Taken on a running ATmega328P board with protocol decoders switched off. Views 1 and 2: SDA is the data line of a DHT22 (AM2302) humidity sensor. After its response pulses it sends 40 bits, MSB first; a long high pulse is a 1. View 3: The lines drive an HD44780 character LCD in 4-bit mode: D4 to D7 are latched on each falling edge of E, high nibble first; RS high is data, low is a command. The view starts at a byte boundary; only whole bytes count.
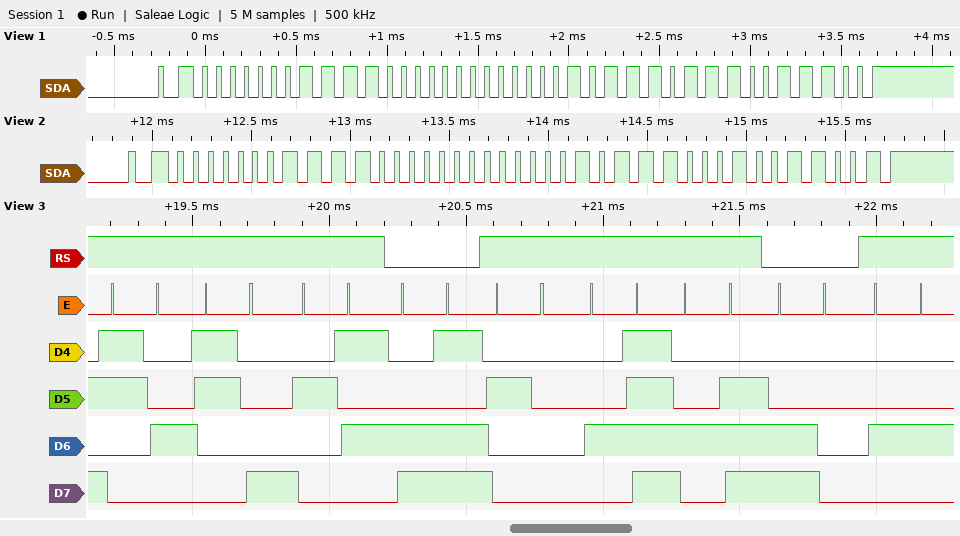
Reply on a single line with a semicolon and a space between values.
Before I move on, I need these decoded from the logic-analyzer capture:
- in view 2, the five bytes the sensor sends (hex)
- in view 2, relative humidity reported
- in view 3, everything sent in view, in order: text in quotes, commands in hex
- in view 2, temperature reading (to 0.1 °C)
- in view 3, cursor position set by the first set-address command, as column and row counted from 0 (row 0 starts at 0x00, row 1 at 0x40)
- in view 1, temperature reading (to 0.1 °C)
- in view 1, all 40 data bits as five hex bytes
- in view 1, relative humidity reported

01 E0 00 B8 99; 48.0 %; "48%" 0xCD " ON" 0xC0 "D"; 18.4 °C; column 13, row 1; 18.7 °C; 01 E0 00 BB 9C; 48.0 %
